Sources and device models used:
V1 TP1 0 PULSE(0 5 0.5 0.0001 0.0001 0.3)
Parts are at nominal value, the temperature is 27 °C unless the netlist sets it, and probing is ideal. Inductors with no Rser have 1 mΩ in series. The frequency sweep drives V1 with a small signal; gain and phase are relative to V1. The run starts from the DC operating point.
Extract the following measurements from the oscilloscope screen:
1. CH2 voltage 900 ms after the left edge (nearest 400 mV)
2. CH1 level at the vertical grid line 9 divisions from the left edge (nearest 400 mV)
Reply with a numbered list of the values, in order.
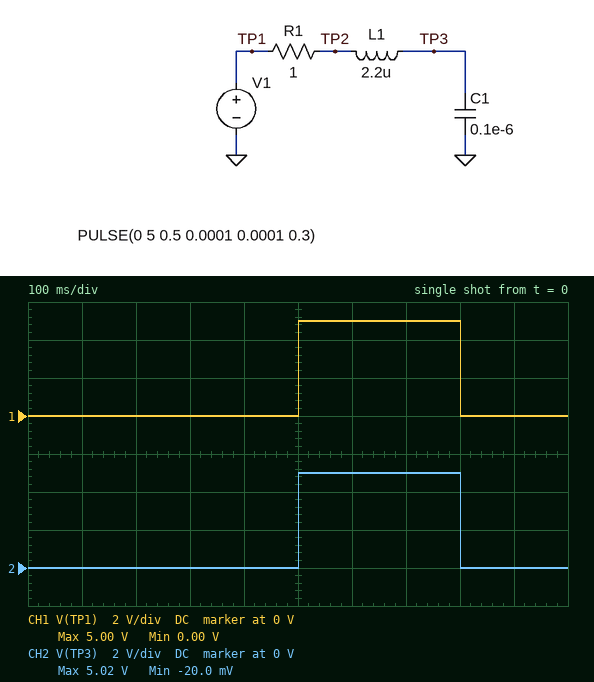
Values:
1. 0 V
2. 0 V
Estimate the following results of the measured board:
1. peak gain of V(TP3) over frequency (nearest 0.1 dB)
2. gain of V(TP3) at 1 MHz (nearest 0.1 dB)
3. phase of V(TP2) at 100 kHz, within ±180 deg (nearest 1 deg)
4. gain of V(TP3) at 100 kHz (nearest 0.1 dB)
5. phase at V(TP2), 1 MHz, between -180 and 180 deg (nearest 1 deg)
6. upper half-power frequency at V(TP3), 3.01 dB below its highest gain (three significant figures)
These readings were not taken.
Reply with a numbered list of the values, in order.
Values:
1. 13.5 dB
2. -17.7 dB
3. -4 deg
4. 0.8 dB
5. 5 deg
6. 370 kHz
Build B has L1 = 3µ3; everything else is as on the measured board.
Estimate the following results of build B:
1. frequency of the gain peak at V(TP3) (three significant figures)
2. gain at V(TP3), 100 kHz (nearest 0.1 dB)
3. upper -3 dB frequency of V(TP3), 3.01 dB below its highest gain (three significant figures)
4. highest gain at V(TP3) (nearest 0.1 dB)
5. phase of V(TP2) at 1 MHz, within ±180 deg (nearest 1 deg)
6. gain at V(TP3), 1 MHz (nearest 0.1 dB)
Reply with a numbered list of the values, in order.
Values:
1. 275 kHz
2. 1.2 dB
3. 298 kHz
4. 15.2 dB
5. 3 deg
6. -21.6 dB
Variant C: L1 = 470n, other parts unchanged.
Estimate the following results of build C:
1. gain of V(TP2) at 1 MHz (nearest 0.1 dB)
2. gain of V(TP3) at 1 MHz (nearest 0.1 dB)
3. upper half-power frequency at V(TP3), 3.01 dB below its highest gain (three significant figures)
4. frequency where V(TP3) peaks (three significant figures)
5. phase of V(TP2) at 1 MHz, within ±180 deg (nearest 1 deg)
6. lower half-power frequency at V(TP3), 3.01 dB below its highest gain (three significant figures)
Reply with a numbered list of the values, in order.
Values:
1. -1.9 dB
2. -0.5 dB
3. 851 kHz
4. 694 kHz
5. 36 deg
6. 489 kHz
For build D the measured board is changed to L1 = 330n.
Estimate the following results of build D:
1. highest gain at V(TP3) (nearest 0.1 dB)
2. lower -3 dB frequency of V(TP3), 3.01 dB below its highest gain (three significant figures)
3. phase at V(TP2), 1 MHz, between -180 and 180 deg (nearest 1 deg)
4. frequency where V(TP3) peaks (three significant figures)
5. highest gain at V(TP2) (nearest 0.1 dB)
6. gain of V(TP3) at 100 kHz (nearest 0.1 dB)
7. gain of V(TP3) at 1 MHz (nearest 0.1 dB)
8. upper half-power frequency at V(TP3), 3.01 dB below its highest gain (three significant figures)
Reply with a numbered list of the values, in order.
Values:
1. 5.5 dB
2. 494 kHz
3. 64 deg
4. 807 kHz
5. 0 dB
6. 0.1 dB
7. 3.1 dB
8. 1.03 MHz
